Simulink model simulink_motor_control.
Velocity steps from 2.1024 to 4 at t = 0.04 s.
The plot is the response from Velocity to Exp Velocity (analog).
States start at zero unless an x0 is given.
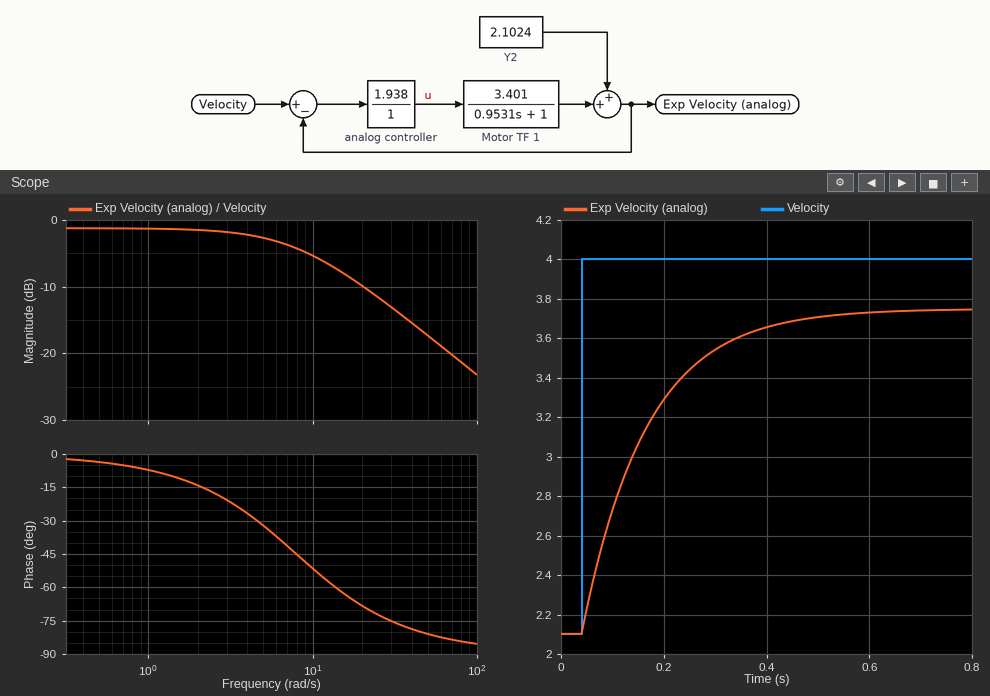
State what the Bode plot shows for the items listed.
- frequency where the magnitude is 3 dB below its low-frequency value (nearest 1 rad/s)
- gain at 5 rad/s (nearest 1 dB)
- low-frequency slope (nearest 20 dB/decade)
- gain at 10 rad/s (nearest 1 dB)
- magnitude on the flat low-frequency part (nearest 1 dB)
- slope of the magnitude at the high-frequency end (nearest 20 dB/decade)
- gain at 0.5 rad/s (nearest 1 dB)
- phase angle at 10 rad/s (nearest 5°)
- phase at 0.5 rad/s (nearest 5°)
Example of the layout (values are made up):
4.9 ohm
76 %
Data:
8 rad/s
-3 dB
0 dB/decade
-5 dB
-1 dB
-20 dB/decade
-1 dB
-50°
-5°
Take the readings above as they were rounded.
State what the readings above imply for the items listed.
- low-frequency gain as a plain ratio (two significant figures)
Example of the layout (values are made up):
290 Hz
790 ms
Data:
0.89
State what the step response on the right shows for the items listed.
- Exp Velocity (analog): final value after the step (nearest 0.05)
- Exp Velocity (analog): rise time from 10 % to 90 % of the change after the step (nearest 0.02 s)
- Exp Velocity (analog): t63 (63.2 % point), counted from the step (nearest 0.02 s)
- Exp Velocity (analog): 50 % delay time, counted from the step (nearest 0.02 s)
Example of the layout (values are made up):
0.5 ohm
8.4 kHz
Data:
3.75
0.28 s
0.12 s
0.08 s
